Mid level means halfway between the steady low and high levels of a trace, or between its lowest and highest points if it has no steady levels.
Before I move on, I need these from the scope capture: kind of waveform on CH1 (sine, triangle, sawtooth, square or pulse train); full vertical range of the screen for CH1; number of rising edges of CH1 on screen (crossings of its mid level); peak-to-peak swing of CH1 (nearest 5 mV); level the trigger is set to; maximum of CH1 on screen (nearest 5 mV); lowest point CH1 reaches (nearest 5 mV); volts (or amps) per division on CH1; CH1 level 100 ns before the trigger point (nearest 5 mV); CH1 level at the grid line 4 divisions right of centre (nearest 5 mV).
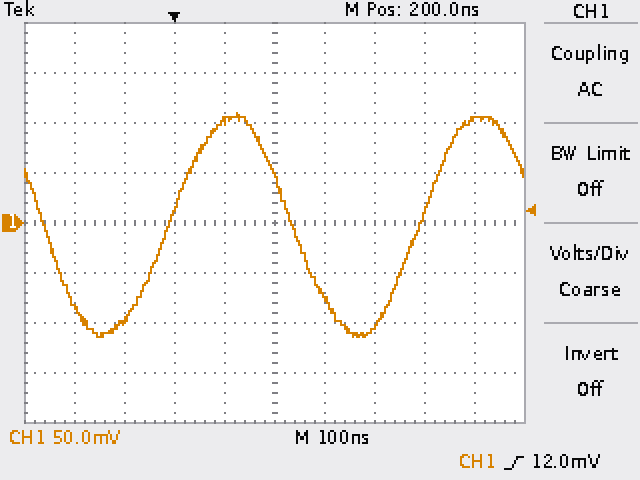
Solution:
sine
400 mV
2
225 mV
12.0 mV
110 mV
-115 mV
50 mV
-95 mV
105 mV
